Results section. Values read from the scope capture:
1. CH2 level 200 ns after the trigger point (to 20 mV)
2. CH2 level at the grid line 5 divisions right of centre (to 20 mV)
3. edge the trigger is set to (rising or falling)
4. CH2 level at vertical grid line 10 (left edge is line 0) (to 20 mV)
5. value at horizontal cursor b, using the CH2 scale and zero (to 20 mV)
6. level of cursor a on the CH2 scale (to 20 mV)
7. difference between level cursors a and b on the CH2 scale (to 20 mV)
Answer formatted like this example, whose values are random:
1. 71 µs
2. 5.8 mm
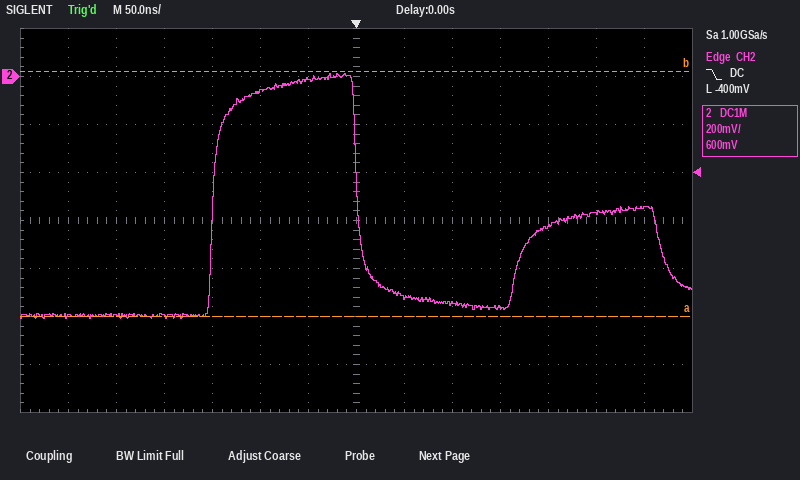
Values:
1. -620 mV
2. -560 mV
3. falling
4. -960 mV
5. 20 mV
6. -1.00 V
7. 1.02 V
